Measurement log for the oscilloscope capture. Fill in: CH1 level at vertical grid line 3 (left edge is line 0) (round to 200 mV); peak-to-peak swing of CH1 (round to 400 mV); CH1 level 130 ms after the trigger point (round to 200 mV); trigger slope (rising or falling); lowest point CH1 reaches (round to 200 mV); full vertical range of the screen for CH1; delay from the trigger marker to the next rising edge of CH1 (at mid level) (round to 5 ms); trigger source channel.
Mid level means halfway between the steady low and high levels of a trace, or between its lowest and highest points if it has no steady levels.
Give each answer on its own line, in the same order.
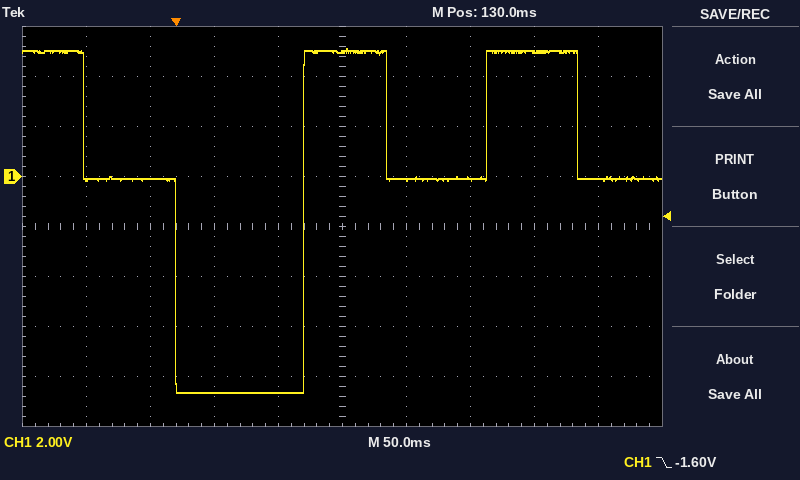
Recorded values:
-8.6 V
13.6 V
5.0 V
falling
-8.6 V
16 V
100 ms
CH1
